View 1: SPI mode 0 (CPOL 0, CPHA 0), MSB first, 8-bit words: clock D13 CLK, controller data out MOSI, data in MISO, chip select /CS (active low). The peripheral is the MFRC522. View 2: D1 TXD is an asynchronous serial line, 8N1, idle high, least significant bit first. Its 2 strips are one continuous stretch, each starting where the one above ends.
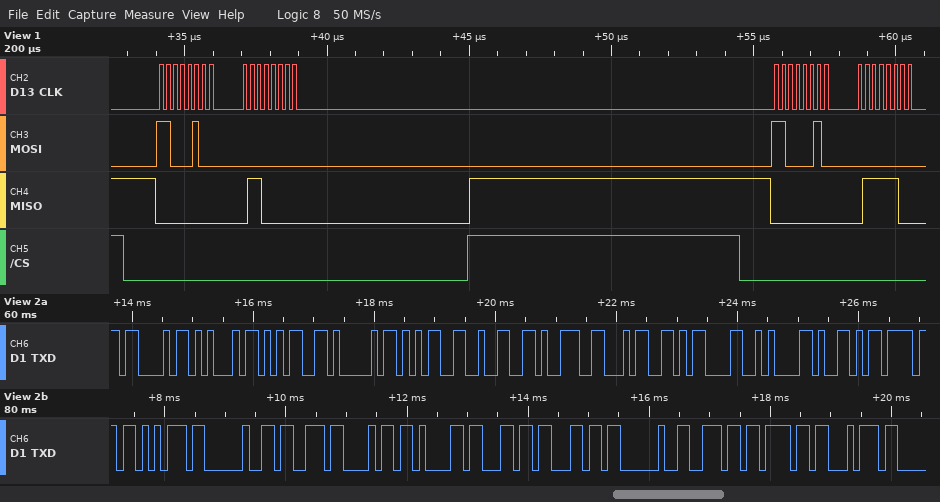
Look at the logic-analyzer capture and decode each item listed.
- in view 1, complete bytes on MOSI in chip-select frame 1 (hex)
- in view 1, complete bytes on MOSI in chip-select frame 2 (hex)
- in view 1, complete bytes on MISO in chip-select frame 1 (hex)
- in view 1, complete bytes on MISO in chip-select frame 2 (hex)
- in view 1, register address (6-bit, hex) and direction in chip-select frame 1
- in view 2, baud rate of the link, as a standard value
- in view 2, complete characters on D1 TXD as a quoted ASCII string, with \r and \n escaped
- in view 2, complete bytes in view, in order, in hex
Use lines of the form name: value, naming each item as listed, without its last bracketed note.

in view 1, complete bytes on MOSI in chip-select frame 1: C4 00
in view 1, complete bytes on MOSI in chip-select frame 2: C2 00
in view 1, complete bytes on MISO in chip-select frame 1: 00 60
in view 1, complete bytes on MISO in chip-select frame 2: 00 7C
in view 1, register address (6-bit, hex) and direction in chip-select frame 1: 0x22 read
in view 2, baud rate of the link, as a standard value: 9600 baud
in view 2, complete characters on D1 TXD as a quoted ASCII string, with \r and \n escaped: "CE5A5294\r\nYou shall not"
in view 2, complete bytes in view, in order, in hex: 43 45 35 41 35 32 39 34 0D 0A 59 6F 75 20 73 68 61 6C 6C 20 6E 6F 74
